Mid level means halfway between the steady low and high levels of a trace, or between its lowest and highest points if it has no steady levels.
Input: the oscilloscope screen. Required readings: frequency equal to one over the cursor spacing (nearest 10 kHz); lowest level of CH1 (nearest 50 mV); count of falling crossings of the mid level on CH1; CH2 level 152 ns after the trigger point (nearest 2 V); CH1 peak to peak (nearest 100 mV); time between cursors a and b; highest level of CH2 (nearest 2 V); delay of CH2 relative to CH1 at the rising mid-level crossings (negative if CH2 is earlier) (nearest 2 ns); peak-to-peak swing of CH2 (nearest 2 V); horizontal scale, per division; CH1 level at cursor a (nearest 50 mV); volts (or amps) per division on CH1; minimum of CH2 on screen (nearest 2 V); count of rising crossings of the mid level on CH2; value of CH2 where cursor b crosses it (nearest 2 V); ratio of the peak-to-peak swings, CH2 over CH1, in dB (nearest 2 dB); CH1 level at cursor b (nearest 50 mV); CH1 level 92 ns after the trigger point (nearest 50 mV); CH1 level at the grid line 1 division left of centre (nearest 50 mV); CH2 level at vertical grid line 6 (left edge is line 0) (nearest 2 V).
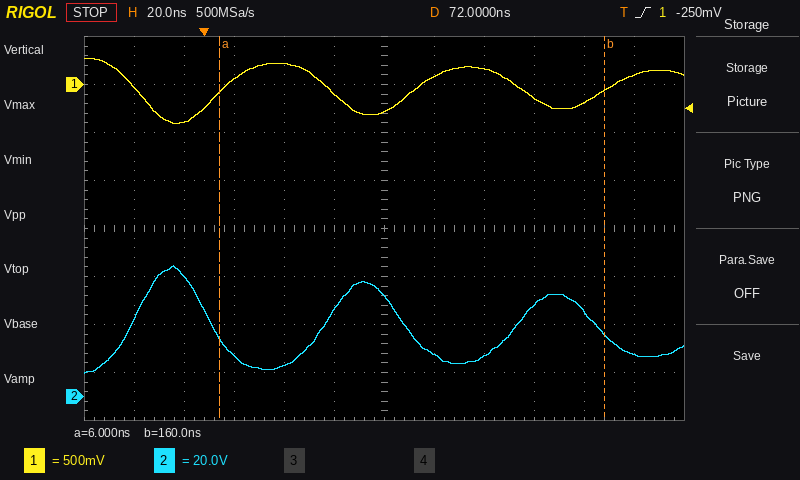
6.49 MHz
-400 mV
3
36 V
700 mV
154 ns
54 V
-34 ns
44 V
20 ns
-100 mV
500 mV
10 V
3
26 V
36 dB
-50 mV
100 mV
-100 mV
42 V
